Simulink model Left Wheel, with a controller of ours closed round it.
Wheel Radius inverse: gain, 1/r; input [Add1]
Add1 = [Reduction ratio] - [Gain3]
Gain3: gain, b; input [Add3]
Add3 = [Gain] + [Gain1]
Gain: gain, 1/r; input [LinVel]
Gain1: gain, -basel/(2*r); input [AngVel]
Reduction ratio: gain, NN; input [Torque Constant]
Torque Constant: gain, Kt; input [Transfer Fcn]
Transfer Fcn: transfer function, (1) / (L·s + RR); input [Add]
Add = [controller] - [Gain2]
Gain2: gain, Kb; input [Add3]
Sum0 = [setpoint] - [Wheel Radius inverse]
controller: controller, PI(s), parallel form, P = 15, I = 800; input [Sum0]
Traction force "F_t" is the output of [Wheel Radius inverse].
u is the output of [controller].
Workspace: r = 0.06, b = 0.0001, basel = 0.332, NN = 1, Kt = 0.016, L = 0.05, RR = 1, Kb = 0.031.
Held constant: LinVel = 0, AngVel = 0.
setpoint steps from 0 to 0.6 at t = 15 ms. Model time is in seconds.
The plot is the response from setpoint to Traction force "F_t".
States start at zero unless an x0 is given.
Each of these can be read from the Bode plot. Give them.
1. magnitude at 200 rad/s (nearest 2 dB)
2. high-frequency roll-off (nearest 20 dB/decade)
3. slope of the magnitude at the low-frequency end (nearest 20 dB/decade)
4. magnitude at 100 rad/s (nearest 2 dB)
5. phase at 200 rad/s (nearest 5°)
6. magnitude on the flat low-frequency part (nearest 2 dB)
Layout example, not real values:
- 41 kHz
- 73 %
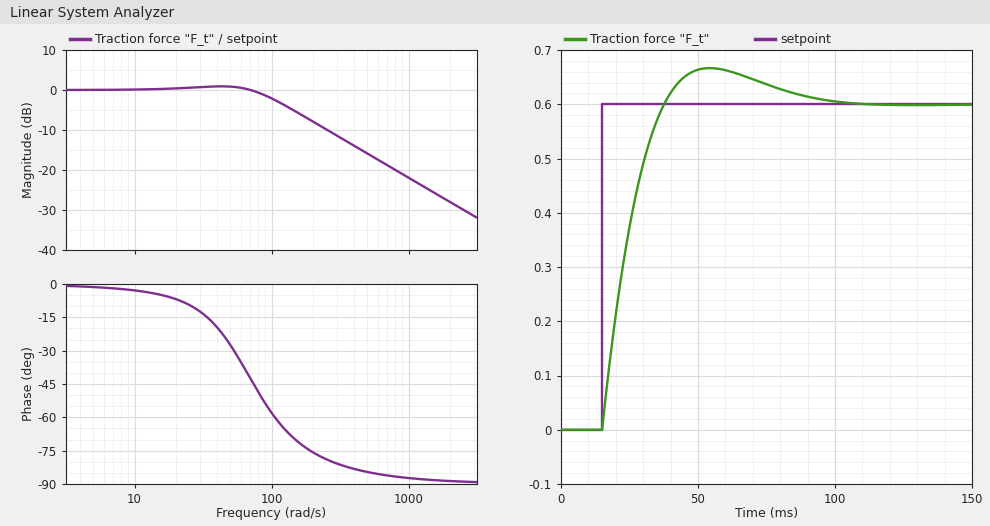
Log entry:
- -8 dB
- -20 dB/decade
- 0 dB/decade
- -2 dB
- -75°
- 0 dB
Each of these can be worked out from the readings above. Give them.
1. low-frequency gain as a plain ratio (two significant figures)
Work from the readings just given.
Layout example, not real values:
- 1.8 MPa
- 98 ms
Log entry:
- 1.0
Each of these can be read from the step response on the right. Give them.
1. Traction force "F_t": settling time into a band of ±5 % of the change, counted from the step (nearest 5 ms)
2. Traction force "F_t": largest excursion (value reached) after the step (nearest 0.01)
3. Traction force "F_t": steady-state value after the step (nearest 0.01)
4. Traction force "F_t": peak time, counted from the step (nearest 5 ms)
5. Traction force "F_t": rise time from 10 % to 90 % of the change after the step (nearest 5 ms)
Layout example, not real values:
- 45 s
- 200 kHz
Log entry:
- 65 ms
- 0.67
- 0.60
- 40 ms
- 15 ms
